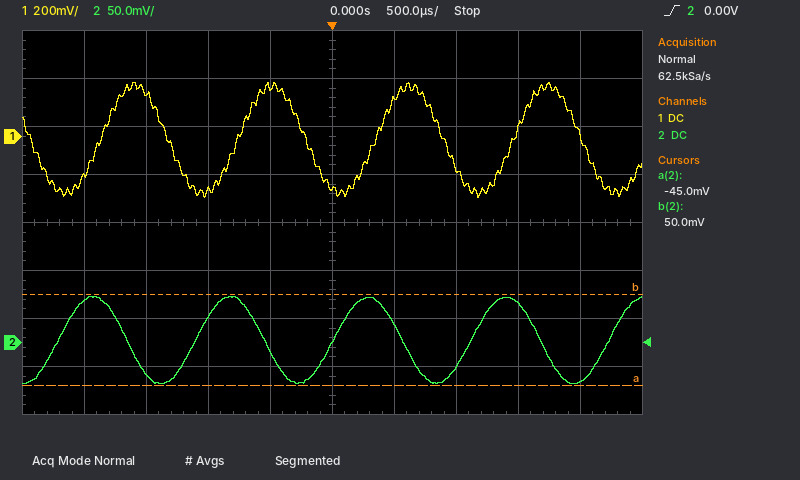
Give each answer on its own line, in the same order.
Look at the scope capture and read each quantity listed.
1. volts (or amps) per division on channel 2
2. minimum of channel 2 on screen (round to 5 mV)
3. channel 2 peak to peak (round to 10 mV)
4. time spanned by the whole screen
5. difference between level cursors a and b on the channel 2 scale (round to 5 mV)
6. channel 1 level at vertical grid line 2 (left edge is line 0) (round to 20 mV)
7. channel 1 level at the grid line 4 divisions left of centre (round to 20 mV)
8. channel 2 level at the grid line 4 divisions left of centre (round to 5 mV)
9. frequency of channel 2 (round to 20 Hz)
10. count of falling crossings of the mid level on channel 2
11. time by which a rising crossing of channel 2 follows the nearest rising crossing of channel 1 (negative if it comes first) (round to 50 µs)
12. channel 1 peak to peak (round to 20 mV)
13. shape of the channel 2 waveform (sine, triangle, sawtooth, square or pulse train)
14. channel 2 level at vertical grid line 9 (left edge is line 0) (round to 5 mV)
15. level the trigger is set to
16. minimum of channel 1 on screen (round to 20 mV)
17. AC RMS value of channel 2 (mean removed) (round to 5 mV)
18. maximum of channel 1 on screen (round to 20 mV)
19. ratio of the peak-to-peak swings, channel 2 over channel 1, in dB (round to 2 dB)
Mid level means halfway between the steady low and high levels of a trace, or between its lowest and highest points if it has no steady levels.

50 mV
-45 mV
90 mV
5 ms
95 mV
180 mV
-160 mV
45 mV
900 Hz
4
-350 µs
480 mV
sine
-40 mV
0.00 V
-260 mV
30 mV
220 mV
-14 dB
